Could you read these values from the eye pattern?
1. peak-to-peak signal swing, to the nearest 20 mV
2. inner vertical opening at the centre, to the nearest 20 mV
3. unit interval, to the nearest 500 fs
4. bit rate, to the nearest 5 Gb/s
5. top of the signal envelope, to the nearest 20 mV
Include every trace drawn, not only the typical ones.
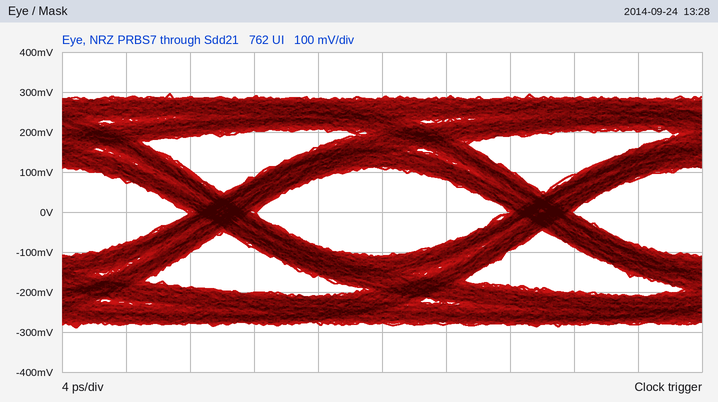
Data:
580 mV
220 mV
20.0 ps
50 Gb/s
300 mV
